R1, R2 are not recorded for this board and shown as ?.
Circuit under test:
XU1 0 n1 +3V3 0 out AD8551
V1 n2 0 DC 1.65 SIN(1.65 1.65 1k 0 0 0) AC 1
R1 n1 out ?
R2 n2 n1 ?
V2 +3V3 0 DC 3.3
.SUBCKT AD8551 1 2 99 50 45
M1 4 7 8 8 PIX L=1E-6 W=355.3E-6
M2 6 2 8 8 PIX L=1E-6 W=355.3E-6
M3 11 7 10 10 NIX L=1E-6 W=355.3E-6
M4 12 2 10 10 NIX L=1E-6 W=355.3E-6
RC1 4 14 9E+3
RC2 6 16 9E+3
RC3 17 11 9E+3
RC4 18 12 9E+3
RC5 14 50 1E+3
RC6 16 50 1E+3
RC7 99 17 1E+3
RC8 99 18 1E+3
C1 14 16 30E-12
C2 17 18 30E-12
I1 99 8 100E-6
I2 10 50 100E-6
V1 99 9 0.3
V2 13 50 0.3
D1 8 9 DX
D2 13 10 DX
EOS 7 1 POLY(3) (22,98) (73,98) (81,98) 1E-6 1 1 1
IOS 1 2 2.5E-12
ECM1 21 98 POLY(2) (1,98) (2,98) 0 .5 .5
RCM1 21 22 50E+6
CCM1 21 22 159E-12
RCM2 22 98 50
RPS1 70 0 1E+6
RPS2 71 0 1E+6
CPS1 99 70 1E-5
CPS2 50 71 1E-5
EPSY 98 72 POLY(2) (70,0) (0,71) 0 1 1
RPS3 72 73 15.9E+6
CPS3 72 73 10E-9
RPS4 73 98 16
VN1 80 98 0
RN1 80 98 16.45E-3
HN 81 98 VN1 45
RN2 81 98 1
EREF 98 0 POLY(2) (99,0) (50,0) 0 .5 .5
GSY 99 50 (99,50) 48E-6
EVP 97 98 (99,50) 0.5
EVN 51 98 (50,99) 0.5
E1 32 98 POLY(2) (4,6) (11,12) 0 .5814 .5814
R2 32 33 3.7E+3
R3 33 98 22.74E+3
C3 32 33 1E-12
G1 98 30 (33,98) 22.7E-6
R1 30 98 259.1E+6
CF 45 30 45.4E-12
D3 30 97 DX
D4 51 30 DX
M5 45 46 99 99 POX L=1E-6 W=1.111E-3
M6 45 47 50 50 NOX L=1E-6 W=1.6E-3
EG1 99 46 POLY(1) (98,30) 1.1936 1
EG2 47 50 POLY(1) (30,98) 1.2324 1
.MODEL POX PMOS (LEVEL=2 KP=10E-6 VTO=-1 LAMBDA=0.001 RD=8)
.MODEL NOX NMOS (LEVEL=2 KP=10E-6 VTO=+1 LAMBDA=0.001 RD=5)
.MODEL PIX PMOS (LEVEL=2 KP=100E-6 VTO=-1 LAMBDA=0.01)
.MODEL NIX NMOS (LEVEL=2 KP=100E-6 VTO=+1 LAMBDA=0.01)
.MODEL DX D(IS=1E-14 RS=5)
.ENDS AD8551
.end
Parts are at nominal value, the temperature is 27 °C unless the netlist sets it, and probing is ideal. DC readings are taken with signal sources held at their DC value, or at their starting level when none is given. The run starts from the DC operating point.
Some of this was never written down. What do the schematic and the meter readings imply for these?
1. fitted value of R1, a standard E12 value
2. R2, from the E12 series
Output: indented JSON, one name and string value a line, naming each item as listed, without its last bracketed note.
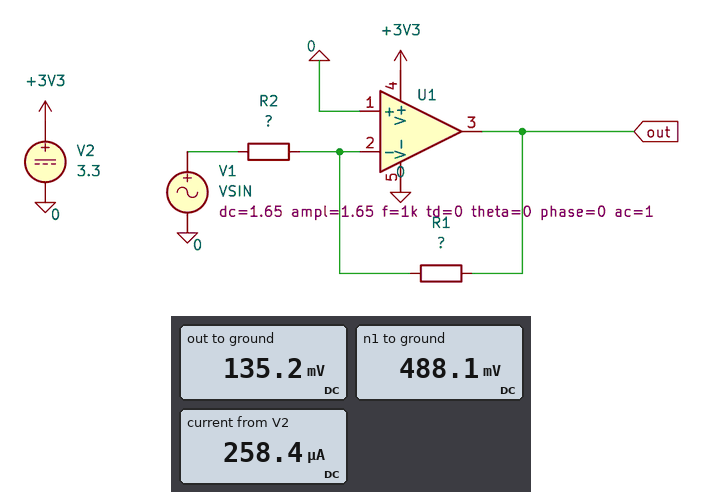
{
  "fitted value of R1, a standard E12 value": "82 Ω",
  "R2, from the E12 series": "270 Ω"
}
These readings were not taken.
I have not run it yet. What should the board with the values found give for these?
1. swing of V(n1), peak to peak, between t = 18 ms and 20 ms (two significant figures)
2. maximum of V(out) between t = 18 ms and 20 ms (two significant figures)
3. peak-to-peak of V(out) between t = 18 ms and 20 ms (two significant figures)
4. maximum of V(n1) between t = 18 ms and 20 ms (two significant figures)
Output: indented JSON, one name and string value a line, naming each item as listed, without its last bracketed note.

{
  "swing of V(n1), peak to peak, between t = 18 ms and 20 ms": "980 mV",
  "maximum of V(out) between t = 18 ms and 20 ms": "270 mV",
  "peak-to-peak of V(out) between t = 18 ms and 20 ms": "270 mV",
  "maximum of V(n1) between t = 18 ms and 20 ms": "980 mV"
}
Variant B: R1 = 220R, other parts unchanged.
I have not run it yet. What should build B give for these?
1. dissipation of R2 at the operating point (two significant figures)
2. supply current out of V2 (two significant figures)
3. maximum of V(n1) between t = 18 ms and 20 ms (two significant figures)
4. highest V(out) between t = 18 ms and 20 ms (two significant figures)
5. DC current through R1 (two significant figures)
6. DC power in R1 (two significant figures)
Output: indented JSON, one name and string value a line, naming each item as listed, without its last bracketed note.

{
  "dissipation of R2 at the operating point": "2.7 mW",
  "supply current out of V2": "330 µA",
  "maximum of V(n1) between t = 18 ms and 20 ms": "1.6 V",
  "highest V(out) between t = 18 ms and 20 ms": "200 mV",
  "DC current through R1": "3.2 mA",
  "DC power in R1": "2.2 mW"
}
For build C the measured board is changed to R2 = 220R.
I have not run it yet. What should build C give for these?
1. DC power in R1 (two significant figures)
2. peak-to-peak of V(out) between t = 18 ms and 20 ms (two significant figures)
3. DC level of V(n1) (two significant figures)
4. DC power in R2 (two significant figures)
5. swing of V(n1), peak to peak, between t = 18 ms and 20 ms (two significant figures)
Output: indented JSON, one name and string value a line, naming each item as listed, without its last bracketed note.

{
  "DC power in R1": "2.0 mW",
  "peak-to-peak of V(out) between t = 18 ms and 20 ms": "320 mV",
  "DC level of V(n1)": "560 mV",
  "DC power in R2": "5.4 mW",
  "swing of V(n1), peak to peak, between t = 18 ms and 20 ms": "1.1 V"
}
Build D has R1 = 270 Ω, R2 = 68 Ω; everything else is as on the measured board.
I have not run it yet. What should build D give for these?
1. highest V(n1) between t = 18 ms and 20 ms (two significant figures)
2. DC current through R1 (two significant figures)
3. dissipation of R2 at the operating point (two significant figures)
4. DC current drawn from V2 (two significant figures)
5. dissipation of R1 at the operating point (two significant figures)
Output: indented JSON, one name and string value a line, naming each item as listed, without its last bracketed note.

{
  "highest V(n1) between t = 18 ms and 20 ms": "2.7 V",
  "DC current through R1": "4.5 mA",
  "dissipation of R2 at the operating point": "1.4 mW",
  "DC current drawn from V2": "360 µA",
  "dissipation of R1 at the operating point": "5.4 mW"
}
